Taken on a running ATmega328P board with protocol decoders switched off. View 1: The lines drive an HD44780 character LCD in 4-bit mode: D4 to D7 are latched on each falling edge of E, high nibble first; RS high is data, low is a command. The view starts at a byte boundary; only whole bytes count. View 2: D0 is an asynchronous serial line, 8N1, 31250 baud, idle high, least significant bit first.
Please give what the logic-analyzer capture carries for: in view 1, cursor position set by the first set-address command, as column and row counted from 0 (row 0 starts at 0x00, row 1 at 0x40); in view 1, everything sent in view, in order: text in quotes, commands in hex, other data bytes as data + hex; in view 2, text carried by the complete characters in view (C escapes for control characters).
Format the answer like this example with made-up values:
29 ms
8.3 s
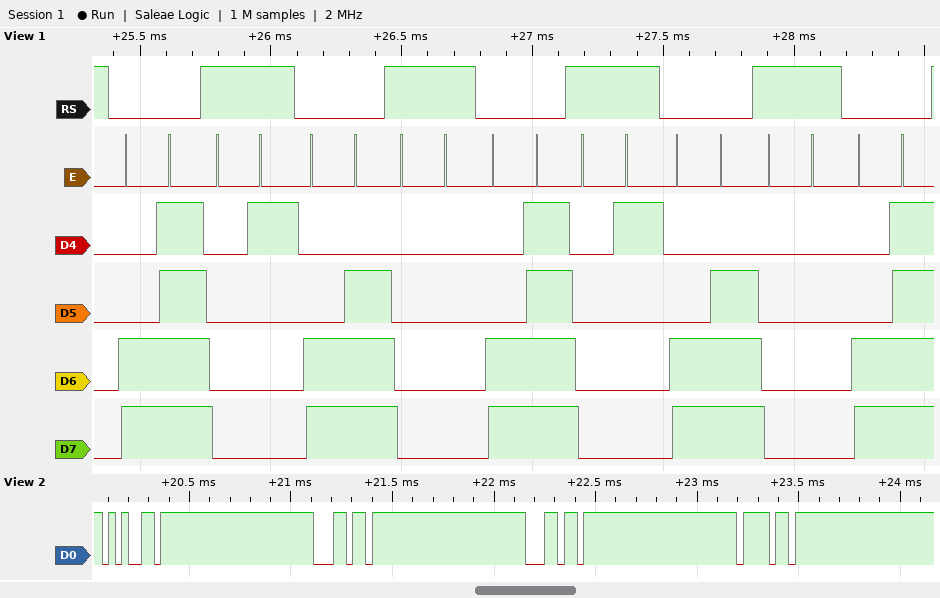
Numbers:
column 15, row 1
0xCF data 01 0xCE data 00 0xCF data 01 0xCE data 00 0xCF
"ello"
